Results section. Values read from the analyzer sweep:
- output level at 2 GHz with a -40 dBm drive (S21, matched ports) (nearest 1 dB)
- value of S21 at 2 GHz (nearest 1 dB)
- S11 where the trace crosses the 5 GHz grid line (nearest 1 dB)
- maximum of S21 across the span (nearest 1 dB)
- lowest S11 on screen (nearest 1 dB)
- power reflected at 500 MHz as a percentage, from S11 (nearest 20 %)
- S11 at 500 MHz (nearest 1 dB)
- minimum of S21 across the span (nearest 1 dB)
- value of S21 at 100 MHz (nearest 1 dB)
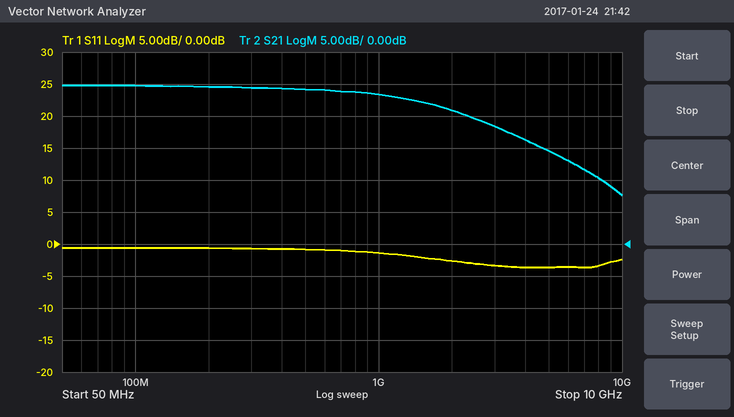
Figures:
-19 dBm
21 dB
-4 dB
25 dB
-4 dB
80 %
-1 dB
8 dB
25 dB
